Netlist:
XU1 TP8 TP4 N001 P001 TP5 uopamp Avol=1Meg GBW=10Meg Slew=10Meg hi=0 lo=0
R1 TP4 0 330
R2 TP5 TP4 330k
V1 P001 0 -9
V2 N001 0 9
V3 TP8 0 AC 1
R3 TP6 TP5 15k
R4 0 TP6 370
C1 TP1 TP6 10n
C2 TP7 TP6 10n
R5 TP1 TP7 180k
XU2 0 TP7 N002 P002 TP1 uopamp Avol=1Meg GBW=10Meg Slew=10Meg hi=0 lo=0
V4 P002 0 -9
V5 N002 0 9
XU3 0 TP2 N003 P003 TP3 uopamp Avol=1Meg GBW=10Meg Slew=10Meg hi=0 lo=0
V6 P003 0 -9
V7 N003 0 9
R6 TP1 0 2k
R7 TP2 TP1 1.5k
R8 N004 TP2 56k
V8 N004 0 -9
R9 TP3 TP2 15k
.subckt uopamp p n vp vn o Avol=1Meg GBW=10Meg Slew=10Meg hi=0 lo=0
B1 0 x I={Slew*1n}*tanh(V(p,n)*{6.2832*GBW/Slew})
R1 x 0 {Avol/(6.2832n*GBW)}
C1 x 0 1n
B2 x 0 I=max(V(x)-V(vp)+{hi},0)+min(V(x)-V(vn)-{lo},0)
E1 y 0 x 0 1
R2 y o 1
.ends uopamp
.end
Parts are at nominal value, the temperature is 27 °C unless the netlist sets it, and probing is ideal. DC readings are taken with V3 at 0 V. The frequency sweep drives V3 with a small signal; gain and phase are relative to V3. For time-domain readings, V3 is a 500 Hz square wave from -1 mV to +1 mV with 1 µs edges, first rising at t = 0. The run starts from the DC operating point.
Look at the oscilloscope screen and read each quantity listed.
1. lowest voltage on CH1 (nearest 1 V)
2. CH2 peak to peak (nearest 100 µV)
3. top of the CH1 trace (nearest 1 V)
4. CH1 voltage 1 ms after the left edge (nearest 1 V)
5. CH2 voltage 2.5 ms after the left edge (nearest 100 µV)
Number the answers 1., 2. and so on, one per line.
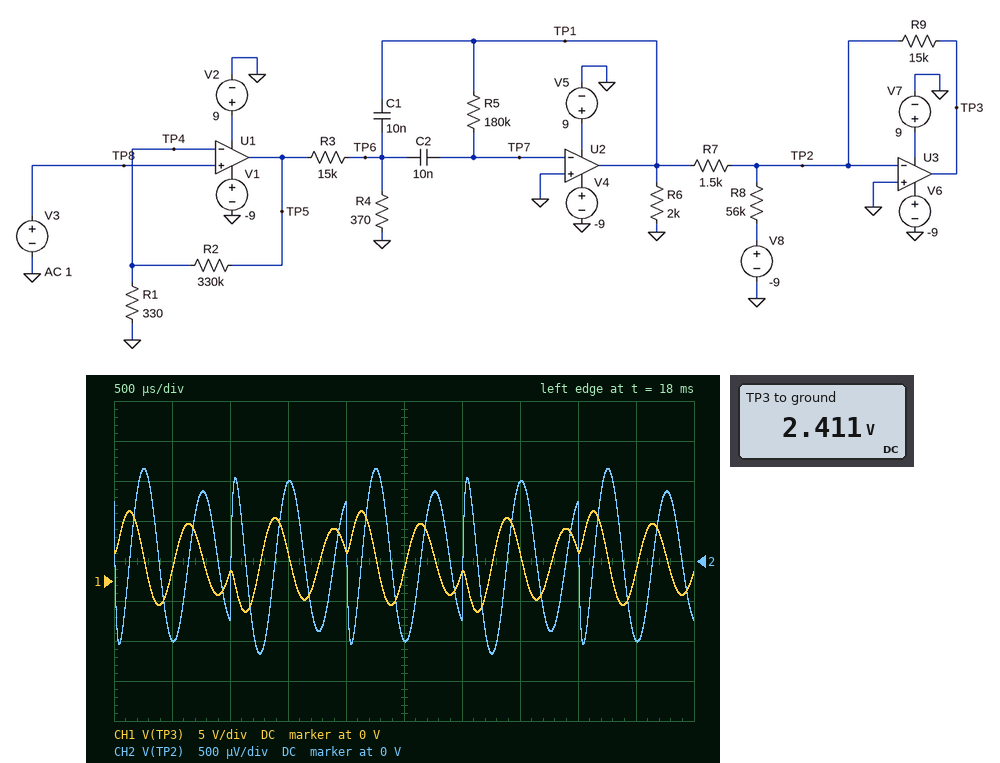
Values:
1. -4 V
2. 2.3 mV
3. 9 V
4. 1 V
5. -1.0 mV
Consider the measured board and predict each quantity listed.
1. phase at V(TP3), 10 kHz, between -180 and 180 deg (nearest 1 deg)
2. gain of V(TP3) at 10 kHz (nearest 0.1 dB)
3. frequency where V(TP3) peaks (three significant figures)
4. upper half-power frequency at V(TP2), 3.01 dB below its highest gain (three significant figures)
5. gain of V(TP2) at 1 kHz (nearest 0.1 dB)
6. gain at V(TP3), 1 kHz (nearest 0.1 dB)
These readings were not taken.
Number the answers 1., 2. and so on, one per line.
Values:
1. -135 deg
2. 57.8 dB
3. 1.97 kHz
4. 2.07 kHz
5. -8.8 dB
6. 71.2 dB
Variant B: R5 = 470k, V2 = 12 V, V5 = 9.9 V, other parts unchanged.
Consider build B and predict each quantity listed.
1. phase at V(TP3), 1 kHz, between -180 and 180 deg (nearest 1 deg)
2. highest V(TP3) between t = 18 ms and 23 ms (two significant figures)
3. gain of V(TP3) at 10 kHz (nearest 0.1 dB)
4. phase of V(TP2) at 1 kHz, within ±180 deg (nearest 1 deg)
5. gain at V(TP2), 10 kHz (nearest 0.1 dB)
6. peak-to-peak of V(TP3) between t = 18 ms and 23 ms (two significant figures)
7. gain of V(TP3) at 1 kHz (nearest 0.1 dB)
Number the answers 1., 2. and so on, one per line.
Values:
1. 76 deg
2. 9.0 V
3. 57.6 dB
4. -14 deg
5. -2.4 dB
6. 18 V
7. 86.6 dB
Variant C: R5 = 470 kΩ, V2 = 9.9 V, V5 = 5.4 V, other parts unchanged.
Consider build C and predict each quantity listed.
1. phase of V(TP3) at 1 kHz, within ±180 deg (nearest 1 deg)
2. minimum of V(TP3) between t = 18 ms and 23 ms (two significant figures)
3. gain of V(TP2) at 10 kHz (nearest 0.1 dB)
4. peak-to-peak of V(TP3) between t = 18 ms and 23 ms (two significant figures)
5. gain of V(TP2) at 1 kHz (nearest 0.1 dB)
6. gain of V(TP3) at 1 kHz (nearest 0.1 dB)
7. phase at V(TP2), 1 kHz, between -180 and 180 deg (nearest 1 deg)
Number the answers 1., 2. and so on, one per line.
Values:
1. 76 deg
2. -9.0 V
3. -2.4 dB
4. 18 V
5. 6.6 dB
6. 86.6 dB
7. -14 deg
